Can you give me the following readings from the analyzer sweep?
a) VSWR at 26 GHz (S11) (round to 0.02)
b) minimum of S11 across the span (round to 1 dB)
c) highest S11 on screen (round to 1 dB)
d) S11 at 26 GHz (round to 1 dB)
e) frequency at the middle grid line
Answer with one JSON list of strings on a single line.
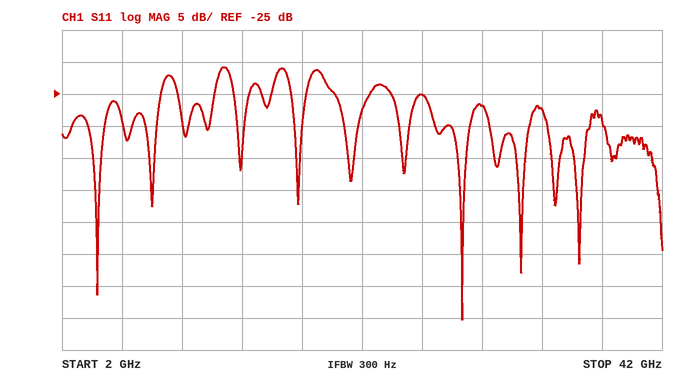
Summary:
["1.12", "-60 dB", "-21 dB", "-25 dB", "22 GHz"]
